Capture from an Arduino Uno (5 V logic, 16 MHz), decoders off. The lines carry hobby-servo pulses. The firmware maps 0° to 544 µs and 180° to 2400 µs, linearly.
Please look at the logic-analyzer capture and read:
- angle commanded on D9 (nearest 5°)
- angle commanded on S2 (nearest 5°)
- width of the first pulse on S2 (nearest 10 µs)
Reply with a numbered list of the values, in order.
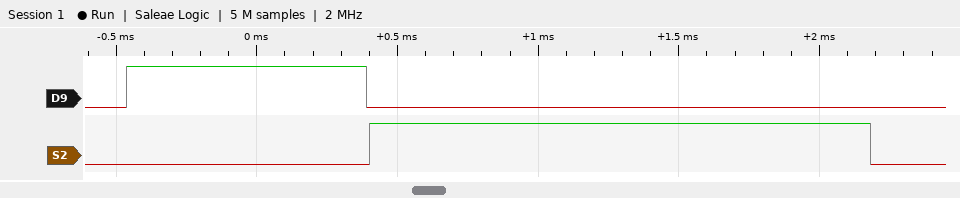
1. 30°
2. 120°
3. 1780 µs
